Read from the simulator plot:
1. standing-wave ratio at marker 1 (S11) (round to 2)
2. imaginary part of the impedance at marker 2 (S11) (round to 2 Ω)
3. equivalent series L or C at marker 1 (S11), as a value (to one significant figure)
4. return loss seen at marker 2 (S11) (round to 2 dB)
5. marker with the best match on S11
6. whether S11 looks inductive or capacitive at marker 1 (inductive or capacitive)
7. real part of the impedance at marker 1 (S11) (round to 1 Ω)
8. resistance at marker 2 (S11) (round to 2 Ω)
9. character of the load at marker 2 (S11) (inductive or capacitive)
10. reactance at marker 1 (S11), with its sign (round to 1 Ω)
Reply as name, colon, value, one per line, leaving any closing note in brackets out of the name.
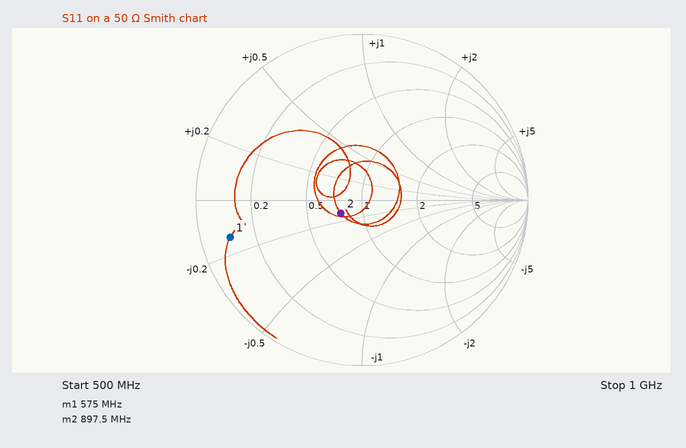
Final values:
standing-wave ratio at marker 1 (S11): 10
imaginary part of the impedance at marker 2 (S11): -6 Ω
equivalent series L or C at marker 1 (S11), as a value: 40 pF
return loss seen at marker 2 (S11): 16 dB
marker with the best match on S11: marker 2
whether S11 looks inductive or capacitive at marker 1: capacitive
real part of the impedance at marker 1 (S11): 5 Ω
resistance at marker 2 (S11): 38 Ω
character of the load at marker 2 (S11): capacitive
reactance at marker 1 (S11), with its sign: -7 Ω
